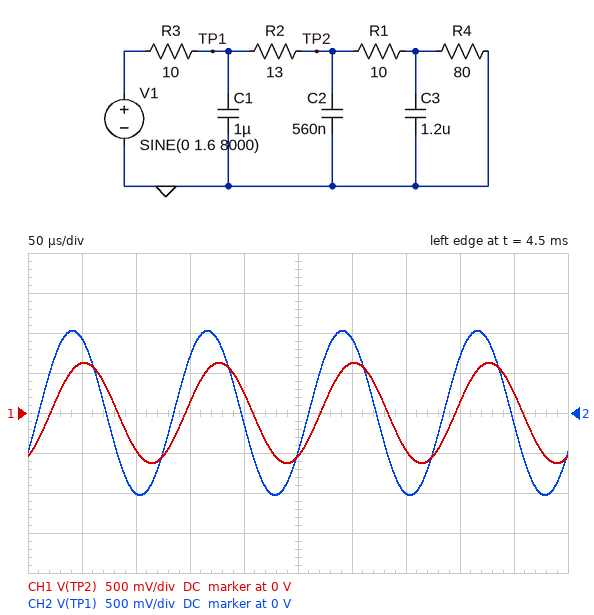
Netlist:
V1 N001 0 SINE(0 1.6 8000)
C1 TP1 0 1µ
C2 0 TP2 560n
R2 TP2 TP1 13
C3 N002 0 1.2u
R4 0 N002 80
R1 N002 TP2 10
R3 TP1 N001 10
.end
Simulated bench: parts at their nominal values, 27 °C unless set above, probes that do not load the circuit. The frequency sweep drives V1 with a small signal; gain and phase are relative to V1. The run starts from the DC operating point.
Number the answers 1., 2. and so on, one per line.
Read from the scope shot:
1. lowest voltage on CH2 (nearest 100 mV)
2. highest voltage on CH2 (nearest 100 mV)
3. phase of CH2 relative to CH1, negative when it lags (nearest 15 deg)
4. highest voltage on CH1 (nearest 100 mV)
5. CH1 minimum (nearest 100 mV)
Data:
1. -1.0 V
2. 1.0 V
3. 30 deg
4. 600 mV
5. -600 mV
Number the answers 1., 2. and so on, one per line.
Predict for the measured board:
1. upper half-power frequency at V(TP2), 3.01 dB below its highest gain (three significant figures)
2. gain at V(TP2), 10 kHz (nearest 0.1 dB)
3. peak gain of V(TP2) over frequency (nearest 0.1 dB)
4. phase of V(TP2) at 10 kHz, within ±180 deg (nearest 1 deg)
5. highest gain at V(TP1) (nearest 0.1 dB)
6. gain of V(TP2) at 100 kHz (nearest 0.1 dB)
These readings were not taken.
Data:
1. 4.33 kHz
2. -9.5 dB
3. -2.0 dB
4. -65 deg
5. -0.8 dB
6. -30.9 dB
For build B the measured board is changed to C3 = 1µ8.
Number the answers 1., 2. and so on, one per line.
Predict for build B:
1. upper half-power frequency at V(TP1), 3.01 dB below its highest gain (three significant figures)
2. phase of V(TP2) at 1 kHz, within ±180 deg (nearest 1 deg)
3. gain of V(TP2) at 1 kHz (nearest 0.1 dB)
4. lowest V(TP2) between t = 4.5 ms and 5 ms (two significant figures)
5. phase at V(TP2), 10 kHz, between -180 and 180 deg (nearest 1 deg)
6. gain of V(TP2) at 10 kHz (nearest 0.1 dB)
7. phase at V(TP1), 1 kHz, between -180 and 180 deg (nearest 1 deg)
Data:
1. 7.37 kHz
2. -16 deg
3. -2.4 dB
4. -550 mV
5. -61 deg
6. -10.5 dB
7. -8 deg
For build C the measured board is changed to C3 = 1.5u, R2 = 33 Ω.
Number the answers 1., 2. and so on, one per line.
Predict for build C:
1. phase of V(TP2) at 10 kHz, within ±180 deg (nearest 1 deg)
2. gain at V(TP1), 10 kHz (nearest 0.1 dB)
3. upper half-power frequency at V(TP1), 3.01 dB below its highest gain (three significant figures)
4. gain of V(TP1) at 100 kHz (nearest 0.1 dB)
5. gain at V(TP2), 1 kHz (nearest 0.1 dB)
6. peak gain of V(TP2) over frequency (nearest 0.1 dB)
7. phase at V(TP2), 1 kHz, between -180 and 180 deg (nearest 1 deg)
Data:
1. -74 deg
2. -3.1 dB
3. 13.2 kHz
4. -16.2 dB
5. -4.0 dB
6. -3.4 dB
7. -21 deg
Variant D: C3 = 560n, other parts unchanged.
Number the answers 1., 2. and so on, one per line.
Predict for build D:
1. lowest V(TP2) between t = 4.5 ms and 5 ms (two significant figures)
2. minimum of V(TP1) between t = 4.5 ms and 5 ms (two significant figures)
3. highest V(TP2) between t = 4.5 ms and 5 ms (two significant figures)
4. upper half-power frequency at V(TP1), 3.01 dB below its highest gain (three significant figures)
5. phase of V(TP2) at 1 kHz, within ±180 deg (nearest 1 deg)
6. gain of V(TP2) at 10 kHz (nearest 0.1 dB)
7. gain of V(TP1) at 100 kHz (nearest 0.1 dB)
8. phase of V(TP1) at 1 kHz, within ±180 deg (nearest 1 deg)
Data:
1. -790 mV
2. -1.1 V
3. 790 mV
4. 9.07 kHz
5. -10 deg
6. -7.5 dB
7. -16.4 dB
8. -6 deg
